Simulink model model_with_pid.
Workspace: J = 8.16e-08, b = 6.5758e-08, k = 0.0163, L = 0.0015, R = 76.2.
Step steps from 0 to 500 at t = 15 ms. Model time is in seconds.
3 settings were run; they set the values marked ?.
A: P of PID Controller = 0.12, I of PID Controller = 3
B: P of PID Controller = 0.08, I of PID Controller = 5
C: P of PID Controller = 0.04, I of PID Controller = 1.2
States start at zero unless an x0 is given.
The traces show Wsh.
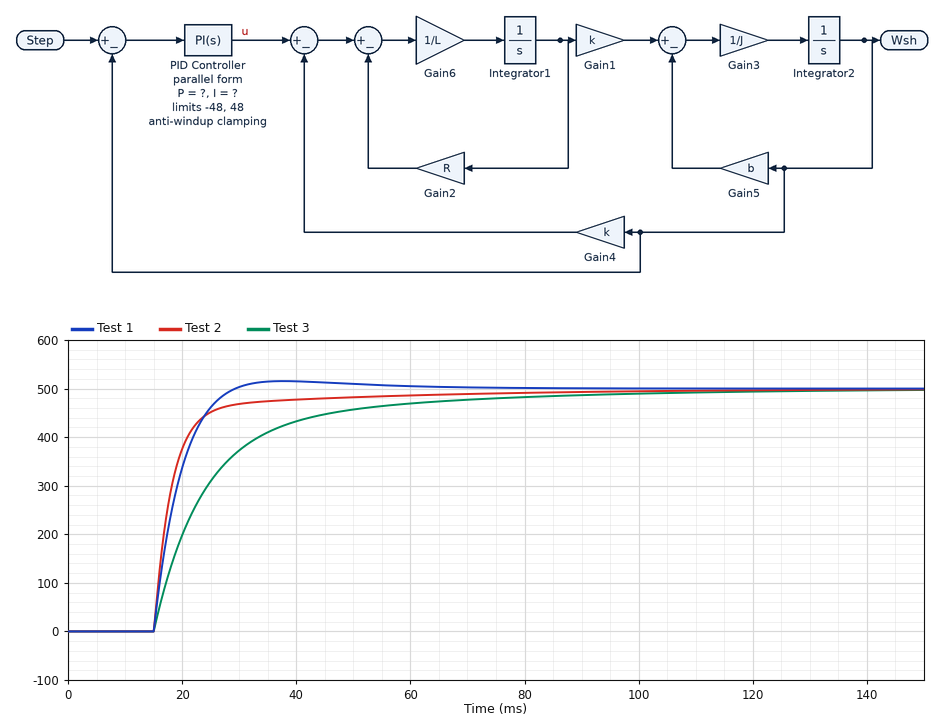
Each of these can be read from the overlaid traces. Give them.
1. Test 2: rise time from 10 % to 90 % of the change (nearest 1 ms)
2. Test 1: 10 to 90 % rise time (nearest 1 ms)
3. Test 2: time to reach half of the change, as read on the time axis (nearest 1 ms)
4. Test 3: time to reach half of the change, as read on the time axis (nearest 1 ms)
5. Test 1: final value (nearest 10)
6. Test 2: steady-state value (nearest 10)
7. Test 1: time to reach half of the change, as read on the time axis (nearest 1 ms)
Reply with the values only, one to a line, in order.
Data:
9 ms
9 ms
17 ms
22 ms
500
500
18 ms
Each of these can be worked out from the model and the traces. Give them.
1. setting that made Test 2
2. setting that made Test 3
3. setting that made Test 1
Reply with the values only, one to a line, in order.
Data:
A
C
B
